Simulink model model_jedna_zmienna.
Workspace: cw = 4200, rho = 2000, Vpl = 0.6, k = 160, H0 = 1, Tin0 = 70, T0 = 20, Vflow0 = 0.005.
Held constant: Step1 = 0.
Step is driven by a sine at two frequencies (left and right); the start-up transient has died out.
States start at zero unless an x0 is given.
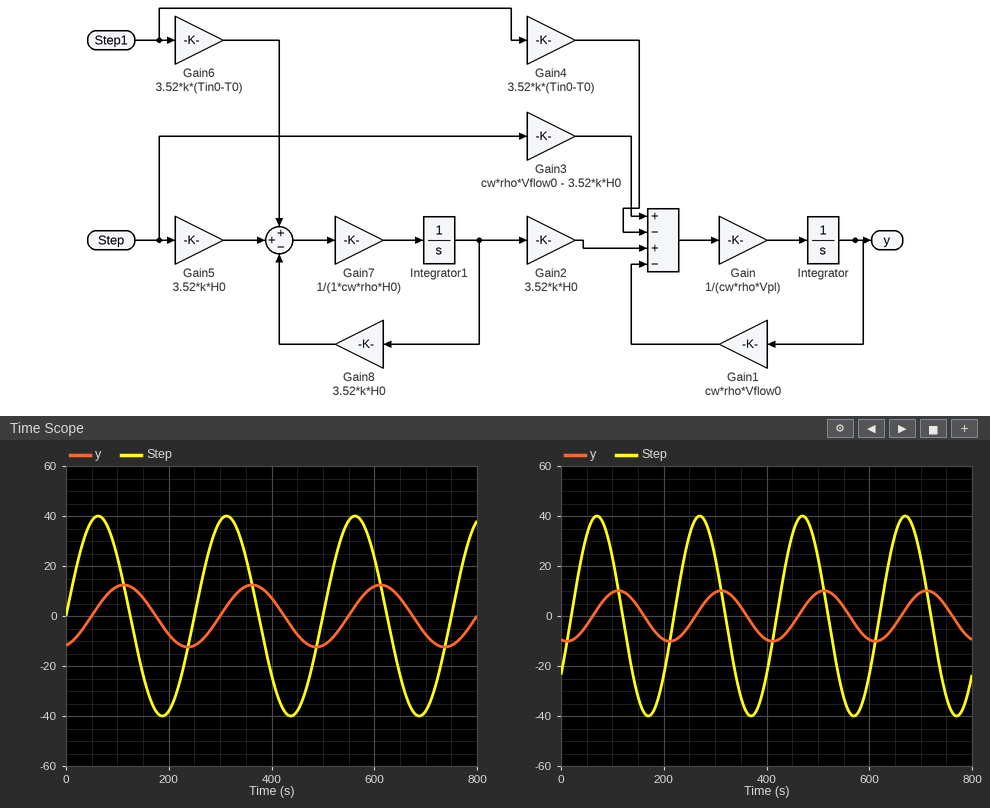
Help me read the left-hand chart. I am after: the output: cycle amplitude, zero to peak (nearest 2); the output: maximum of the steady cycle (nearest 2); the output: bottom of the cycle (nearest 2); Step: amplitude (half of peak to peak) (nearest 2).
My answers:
12
12
-12
40
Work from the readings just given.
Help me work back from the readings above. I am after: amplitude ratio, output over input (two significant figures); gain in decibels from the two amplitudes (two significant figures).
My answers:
0.30
-10 dB
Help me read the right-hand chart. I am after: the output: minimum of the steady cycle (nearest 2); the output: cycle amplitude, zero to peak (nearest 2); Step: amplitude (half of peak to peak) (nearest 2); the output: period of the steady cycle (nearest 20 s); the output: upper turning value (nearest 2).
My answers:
-10
10
40
200 s
10
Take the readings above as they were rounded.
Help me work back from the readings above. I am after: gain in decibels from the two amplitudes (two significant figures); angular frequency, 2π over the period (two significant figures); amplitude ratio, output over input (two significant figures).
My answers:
-12 dB
0.031 rad/s
0.25
